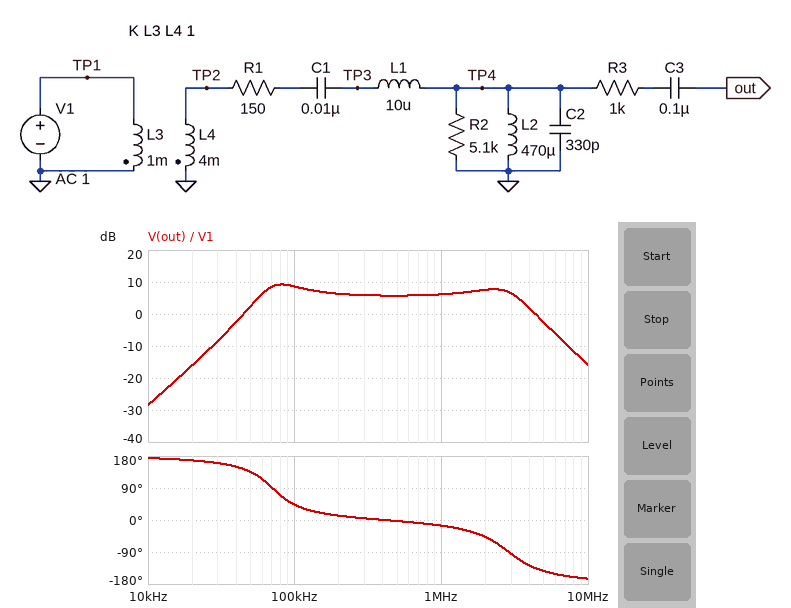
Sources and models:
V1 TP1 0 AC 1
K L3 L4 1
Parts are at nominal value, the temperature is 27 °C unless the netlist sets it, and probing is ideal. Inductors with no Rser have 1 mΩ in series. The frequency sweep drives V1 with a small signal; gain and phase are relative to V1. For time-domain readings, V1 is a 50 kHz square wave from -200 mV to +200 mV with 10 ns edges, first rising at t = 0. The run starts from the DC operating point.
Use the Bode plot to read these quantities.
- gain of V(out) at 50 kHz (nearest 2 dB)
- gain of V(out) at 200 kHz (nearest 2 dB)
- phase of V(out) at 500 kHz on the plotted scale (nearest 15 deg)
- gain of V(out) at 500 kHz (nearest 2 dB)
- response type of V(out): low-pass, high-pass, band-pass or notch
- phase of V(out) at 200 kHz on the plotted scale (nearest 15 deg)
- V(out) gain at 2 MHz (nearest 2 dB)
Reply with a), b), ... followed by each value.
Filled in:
a) 2 dB
b) 6 dB
c) 0 deg
d) 6 dB
e) band-pass
f) 15 deg
g) 8 dB
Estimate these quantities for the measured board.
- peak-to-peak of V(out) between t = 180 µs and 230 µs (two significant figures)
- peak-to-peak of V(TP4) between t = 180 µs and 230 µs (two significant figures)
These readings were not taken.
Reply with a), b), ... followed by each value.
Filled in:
a) 1.8 V
b) 1.8 V
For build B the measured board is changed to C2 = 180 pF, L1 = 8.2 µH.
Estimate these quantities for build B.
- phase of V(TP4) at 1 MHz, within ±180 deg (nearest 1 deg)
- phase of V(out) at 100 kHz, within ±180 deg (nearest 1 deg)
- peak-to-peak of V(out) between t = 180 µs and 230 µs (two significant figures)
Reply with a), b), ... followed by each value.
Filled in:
a) -7 deg
b) 45 deg
c) 1.9 V
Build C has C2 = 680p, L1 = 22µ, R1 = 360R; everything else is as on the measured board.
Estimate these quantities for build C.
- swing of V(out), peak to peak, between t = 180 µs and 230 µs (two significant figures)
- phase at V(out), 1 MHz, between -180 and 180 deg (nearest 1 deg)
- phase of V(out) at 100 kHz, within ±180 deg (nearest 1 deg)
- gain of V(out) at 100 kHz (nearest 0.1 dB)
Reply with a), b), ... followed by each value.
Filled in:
a) 1.2 V
b) -68 deg
c) 60 deg
d) 4.0 dB
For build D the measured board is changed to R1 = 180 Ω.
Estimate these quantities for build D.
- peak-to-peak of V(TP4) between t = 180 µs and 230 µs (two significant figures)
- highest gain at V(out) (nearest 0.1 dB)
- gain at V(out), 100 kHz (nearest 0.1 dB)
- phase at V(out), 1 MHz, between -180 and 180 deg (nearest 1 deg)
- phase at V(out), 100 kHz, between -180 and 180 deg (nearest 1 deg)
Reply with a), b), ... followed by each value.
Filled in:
a) 1.7 V
b) 8.0 dB
c) 7.8 dB
d) -19 deg
e) 48 deg
